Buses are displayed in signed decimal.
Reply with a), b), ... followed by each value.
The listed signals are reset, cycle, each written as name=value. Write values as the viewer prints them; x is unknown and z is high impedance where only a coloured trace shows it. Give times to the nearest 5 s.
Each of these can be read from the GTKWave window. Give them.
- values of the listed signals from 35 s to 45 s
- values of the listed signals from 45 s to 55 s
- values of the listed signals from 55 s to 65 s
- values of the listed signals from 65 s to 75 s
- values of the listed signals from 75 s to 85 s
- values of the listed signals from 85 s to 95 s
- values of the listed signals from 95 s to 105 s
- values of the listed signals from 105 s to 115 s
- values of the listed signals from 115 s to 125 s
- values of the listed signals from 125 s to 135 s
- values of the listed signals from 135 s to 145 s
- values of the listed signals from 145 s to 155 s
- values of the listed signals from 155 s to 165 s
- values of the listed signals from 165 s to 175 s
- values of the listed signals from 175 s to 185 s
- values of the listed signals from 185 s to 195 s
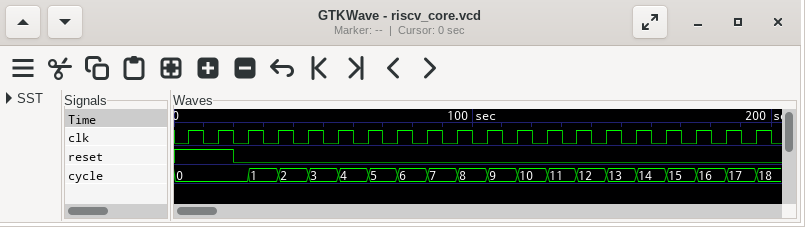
a) reset=0, cycle=2
b) reset=0, cycle=3
c) reset=0, cycle=4
d) reset=0, cycle=5
e) reset=0, cycle=6
f) reset=0, cycle=7
g) reset=0, cycle=8
h) reset=0, cycle=9
i) reset=0, cycle=10
j) reset=0, cycle=11
k) reset=0, cycle=12
l) reset=0, cycle=13
m) reset=0, cycle=14
n) reset=0, cycle=15
o) reset=0, cycle=16
p) reset=0, cycle=17
